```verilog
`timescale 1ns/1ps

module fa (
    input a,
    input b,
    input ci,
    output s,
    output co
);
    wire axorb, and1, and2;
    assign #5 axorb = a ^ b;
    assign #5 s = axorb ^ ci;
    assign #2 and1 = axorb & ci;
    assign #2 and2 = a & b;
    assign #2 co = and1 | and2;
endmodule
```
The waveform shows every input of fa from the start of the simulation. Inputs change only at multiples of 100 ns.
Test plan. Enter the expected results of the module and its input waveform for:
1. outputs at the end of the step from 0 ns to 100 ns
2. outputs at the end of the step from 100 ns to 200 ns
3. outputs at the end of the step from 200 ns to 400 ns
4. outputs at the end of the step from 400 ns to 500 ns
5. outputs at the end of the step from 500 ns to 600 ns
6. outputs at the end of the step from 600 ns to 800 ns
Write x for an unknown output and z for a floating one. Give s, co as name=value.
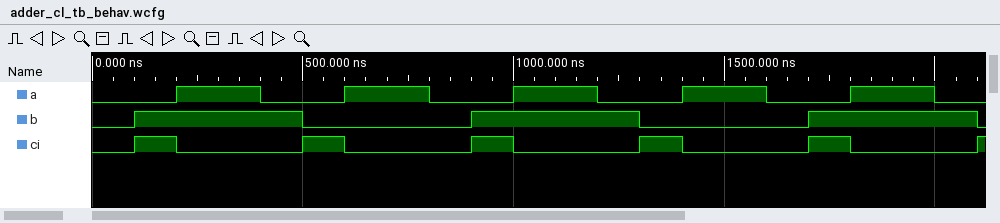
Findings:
s=0, co=0
s=0, co=1
s=0, co=1
s=1, co=0
s=1, co=0
s=1, co=0
